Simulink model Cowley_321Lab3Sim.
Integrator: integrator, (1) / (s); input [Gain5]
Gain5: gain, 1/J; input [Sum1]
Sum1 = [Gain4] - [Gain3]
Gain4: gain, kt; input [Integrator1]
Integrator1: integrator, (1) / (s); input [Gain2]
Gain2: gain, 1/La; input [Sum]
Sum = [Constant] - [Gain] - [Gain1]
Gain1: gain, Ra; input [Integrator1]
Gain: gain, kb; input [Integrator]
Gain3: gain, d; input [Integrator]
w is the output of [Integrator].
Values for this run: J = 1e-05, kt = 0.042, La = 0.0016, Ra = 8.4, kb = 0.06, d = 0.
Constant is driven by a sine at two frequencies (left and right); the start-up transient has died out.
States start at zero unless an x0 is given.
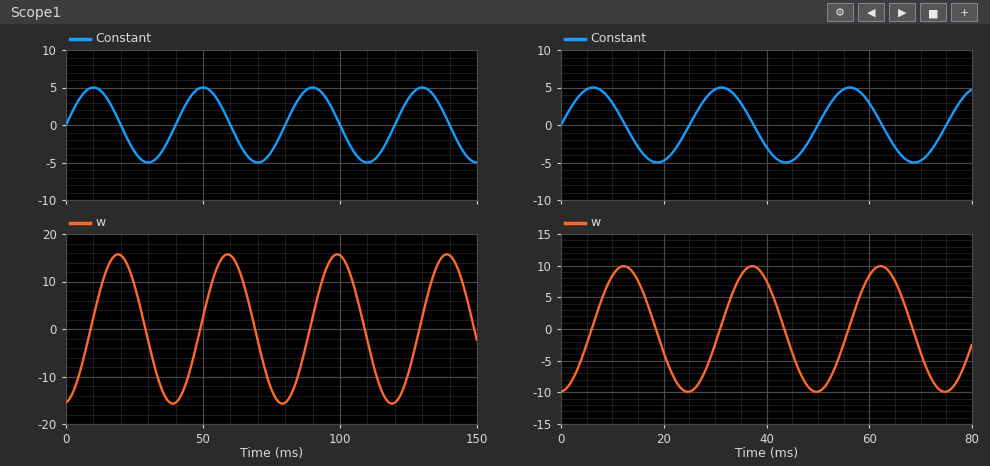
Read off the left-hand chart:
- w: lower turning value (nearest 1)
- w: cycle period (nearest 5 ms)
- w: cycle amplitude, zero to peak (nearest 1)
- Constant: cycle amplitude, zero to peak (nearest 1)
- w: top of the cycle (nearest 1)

-16
40 ms
16
5
16
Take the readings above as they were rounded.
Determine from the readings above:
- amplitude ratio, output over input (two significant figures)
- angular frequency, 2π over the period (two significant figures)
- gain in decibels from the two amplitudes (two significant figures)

3.2
0.16 rad/ms
10 dB
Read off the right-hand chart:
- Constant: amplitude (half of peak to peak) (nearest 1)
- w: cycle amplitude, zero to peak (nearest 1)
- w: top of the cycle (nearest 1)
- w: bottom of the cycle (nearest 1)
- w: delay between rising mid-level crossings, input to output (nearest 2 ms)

5
10
10
-10
6 ms
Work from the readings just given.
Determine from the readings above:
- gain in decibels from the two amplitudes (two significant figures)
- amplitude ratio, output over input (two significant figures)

6.0 dB
2.0
